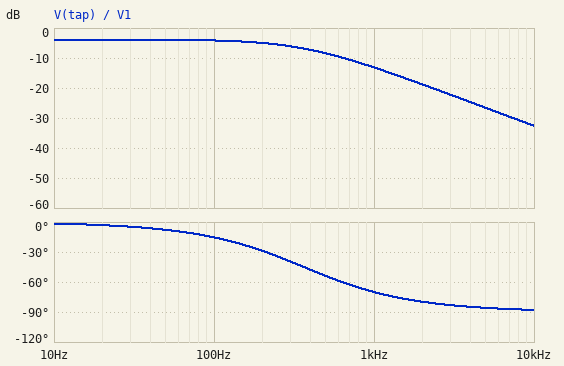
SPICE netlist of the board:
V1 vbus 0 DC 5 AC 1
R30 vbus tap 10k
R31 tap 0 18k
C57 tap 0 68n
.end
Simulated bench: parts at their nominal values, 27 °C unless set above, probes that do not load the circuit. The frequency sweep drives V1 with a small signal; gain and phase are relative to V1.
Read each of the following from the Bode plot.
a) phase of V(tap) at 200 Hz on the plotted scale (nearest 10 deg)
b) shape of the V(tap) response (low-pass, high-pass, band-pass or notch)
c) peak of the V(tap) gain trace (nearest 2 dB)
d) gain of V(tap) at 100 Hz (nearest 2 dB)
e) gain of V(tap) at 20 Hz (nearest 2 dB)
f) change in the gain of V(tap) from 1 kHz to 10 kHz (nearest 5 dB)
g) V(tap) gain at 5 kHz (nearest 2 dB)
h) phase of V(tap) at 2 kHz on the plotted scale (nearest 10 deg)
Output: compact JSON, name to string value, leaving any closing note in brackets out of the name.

{"phase of V(tap) at 200 Hz on the plotted scale": "-30 deg", "shape of the V(tap) response": "low-pass", "peak of the V(tap) gain trace": "-4 dB", "gain of V(tap) at 100 Hz": "-4 dB", "gain of V(tap) at 20 Hz": "-4 dB", "change in the gain of V(tap) from 1 kHz to 10 kHz": "-20 dB", "V(tap) gain at 5 kHz": "-26 dB", "phase of V(tap) at 2 kHz on the plotted scale": "-80 deg"}
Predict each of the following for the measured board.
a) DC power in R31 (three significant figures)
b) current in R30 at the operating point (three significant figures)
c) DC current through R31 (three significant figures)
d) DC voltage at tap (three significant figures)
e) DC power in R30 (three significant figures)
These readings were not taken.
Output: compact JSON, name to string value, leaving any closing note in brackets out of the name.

{"DC power in R31": "574 µW", "current in R30 at the operating point": "179 µA", "DC current through R31": "179 µA", "DC voltage at tap": "3.21 V", "DC power in R30": "319 µW"}
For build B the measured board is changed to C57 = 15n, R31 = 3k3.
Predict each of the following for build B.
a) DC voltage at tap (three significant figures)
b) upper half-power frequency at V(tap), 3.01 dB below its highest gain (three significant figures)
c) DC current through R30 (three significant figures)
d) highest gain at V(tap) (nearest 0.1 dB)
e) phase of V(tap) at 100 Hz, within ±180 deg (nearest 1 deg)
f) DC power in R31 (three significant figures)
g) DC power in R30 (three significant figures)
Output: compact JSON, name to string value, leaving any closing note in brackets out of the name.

{"DC voltage at tap": "1.24 V", "upper half-power frequency at V(tap), 3.01 dB below its highest gain": "4.28 kHz", "DC current through R30": "376 µA", "highest gain at V(tap)": "-12.1 dB", "phase of V(tap) at 100 Hz, within ±180 deg": "-1 deg", "DC power in R31": "466 µW", "DC power in R30": "1.41 mW"}
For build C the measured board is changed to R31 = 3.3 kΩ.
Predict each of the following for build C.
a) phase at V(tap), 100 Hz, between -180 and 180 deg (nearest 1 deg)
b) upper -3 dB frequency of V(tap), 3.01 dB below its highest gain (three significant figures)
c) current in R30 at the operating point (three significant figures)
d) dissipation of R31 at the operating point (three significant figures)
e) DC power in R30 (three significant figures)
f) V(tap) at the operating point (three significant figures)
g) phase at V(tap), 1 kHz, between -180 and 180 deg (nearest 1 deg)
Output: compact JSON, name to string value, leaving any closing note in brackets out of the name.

{"phase at V(tap), 100 Hz, between -180 and 180 deg": "-6 deg", "upper -3 dB frequency of V(tap), 3.01 dB below its highest gain": "943 Hz", "current in R30 at the operating point": "376 µA", "dissipation of R31 at the operating point": "466 µW", "DC power in R30": "1.41 mW", "V(tap) at the operating point": "1.24 V", "phase at V(tap), 1 kHz, between -180 and 180 deg": "-47 deg"}
